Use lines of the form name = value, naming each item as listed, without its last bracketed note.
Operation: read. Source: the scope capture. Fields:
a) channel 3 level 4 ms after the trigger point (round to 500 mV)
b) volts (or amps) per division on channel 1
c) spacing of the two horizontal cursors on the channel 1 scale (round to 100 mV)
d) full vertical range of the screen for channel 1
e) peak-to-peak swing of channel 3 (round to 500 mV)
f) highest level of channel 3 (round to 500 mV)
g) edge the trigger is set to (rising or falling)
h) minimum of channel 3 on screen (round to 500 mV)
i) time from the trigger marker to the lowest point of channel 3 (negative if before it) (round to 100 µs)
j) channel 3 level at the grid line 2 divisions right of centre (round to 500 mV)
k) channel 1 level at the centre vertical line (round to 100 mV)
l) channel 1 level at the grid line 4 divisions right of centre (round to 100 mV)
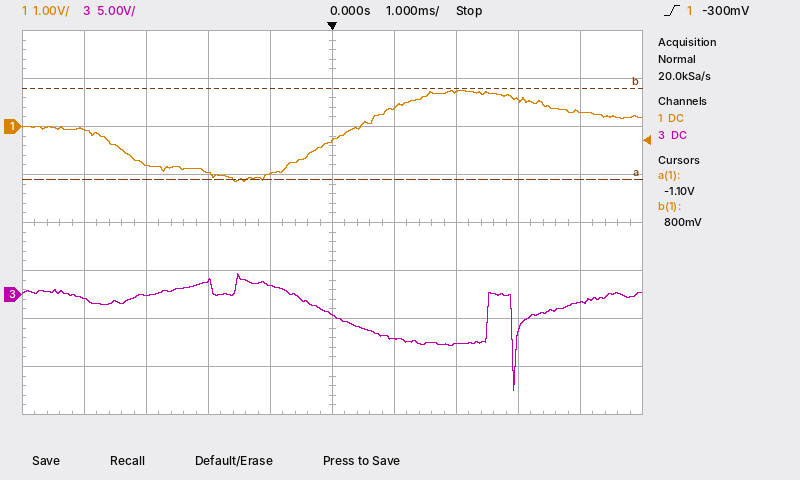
channel 3 level 4 ms after the trigger point = -1.0 V
volts (or amps) per division on channel 1 = 1 V
spacing of the two horizontal cursors on the channel 1 scale = 1.9 V
full vertical range of the screen for channel 1 = 8 V
peak-to-peak swing of channel 3 = 12.0 V
highest level of channel 3 = 2.0 V
edge the trigger is set to = rising
minimum of channel 3 on screen = -10.0 V
time from the trigger marker to the lowest point of channel 3 (negative if before it) = +2.9 ms
channel 3 level at the grid line 2 divisions right of centre = -5.0 V
channel 1 level at the centre vertical line = -300 mV
channel 1 level at the grid line 4 divisions right of centre = 300 mV
